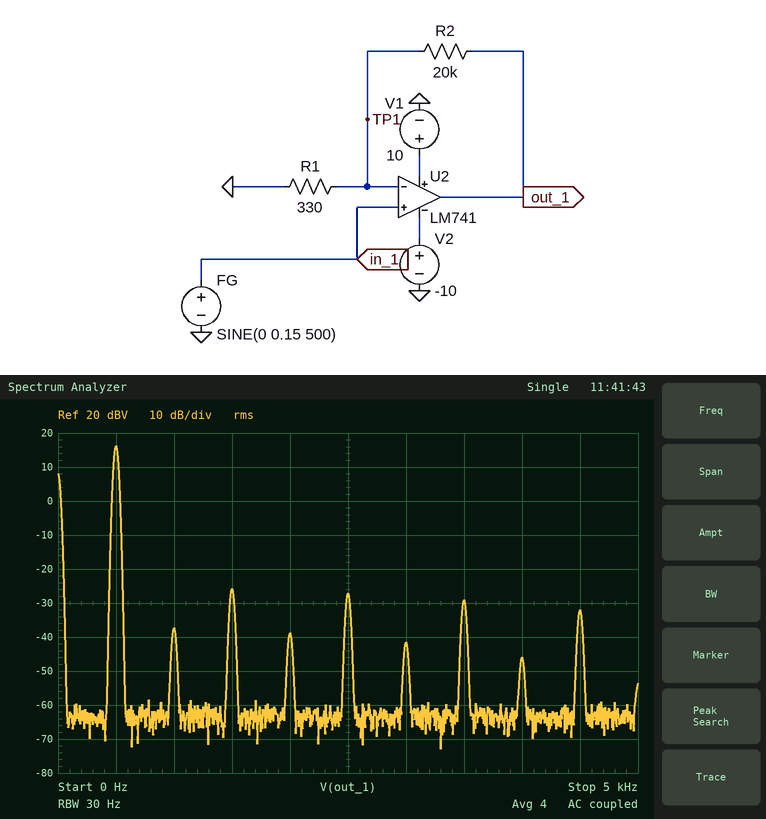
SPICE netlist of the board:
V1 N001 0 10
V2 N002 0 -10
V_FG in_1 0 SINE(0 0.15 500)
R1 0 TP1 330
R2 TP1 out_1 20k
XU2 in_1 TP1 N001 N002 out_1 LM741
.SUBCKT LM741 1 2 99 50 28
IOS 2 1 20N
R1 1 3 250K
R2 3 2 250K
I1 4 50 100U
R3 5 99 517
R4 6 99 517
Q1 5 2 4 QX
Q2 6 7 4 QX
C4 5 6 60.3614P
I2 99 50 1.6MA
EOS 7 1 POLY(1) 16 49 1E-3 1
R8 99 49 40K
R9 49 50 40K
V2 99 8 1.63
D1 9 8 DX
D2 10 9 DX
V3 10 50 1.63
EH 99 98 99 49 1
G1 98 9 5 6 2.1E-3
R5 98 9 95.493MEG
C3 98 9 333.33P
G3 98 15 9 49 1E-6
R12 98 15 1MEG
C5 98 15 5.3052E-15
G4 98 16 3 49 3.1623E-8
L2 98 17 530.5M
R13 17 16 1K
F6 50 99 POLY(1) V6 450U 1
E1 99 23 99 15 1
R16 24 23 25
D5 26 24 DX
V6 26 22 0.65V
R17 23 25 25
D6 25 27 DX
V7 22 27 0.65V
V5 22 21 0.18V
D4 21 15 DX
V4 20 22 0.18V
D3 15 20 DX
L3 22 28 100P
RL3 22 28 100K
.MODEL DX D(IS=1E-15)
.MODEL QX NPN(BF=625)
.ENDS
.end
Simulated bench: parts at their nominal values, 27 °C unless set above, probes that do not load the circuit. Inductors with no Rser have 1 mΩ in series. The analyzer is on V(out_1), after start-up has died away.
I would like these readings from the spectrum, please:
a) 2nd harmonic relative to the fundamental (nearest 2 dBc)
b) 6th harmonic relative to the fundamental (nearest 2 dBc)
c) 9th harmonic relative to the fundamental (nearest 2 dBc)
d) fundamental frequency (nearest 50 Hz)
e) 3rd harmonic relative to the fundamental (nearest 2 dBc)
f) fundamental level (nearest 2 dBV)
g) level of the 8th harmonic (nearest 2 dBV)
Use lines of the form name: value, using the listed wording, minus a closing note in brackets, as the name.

2nd harmonic relative to the fundamental: -54 dBc
6th harmonic relative to the fundamental: -58 dBc
9th harmonic relative to the fundamental: -48 dBc
fundamental frequency: 500 Hz
3rd harmonic relative to the fundamental: -42 dBc
fundamental level: 16 dBV
level of the 8th harmonic: -46 dBV
